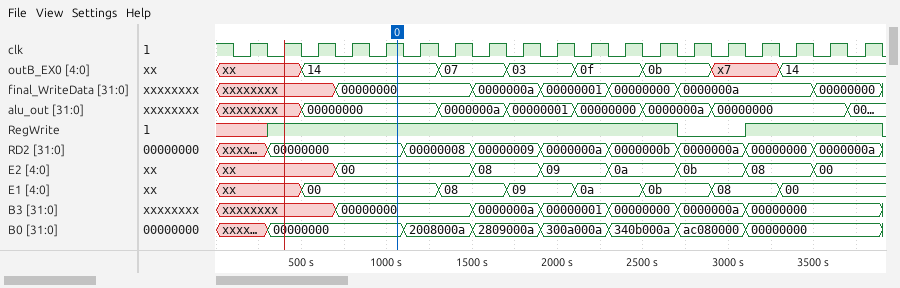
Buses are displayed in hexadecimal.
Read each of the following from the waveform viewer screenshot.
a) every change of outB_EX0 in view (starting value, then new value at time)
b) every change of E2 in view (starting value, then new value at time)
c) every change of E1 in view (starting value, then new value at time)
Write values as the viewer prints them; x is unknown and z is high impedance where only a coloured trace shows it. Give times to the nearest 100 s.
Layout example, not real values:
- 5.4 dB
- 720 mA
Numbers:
- xx, 14 at 500 s, 07 at 1300 s, 03 at 1700 s, 0f at 2100 s, 0b at 2500 s, x7 at 2900 s, 14 at 3300 s
- xx, 00 at 700 s, 08 at 1500 s, 09 at 1900 s, 0a at 2300 s, 0b at 2700 s, 08 at 3100 s, 00 at 3500 s
- xx, 00 at 500 s, 08 at 1300 s, 09 at 1700 s, 0a at 2100 s, 0b at 2500 s, 08 at 2900 s, 00 at 3300 s
